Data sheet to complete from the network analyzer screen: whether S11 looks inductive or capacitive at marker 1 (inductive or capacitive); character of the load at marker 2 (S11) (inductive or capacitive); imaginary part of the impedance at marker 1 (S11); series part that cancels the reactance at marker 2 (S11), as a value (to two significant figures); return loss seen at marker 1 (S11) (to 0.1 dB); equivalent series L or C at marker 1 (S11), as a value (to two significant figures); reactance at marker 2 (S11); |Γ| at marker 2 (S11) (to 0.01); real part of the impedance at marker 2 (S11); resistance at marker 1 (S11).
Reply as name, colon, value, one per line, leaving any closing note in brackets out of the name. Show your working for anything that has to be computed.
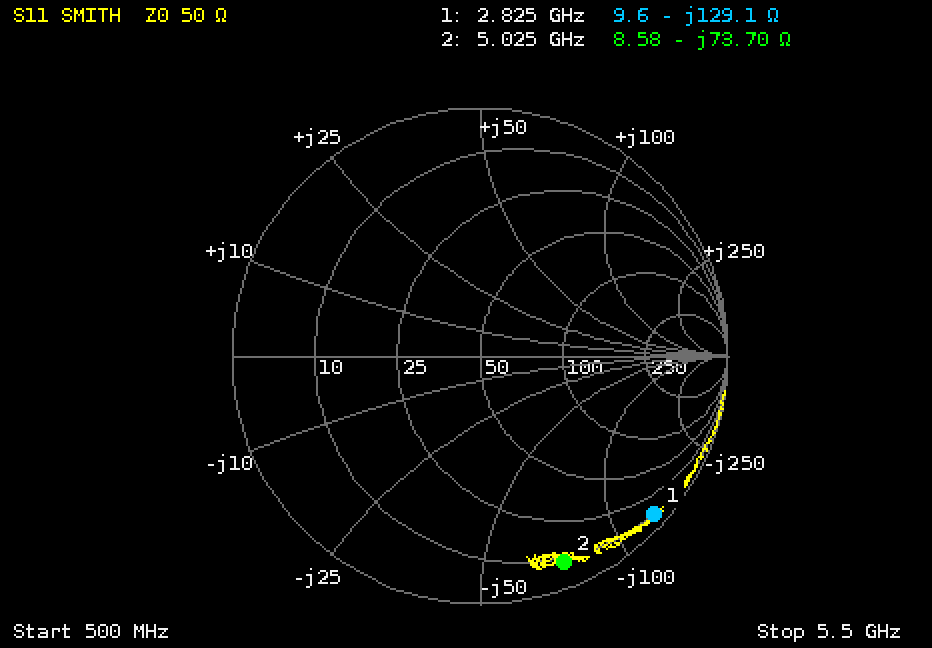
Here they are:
whether S11 looks inductive or capacitive at marker 1: capacitive
character of the load at marker 2 (S11): capacitive
imaginary part of the impedance at marker 1: -129.1 Ω
series part that cancels the reactance at marker 2 (S11), as a value: L = 73.7 Ω/(2π × 5.025 GHz) ≈ 2.3 nH
return loss seen at marker 1 (S11): 0.4 dB
equivalent series L or C at marker 1 (S11), as a value: C = 1/(2π × 2.825 GHz × 129.1 Ω) ≈ 436 fF, so 440 fF to two significant figures
reactance at marker 2: -73.70 Ω
|Γ| at marker 2 (S11): 0.90
real part of the impedance at marker 2: 8.58 Ω
resistance at marker 1: 9.6 Ω
